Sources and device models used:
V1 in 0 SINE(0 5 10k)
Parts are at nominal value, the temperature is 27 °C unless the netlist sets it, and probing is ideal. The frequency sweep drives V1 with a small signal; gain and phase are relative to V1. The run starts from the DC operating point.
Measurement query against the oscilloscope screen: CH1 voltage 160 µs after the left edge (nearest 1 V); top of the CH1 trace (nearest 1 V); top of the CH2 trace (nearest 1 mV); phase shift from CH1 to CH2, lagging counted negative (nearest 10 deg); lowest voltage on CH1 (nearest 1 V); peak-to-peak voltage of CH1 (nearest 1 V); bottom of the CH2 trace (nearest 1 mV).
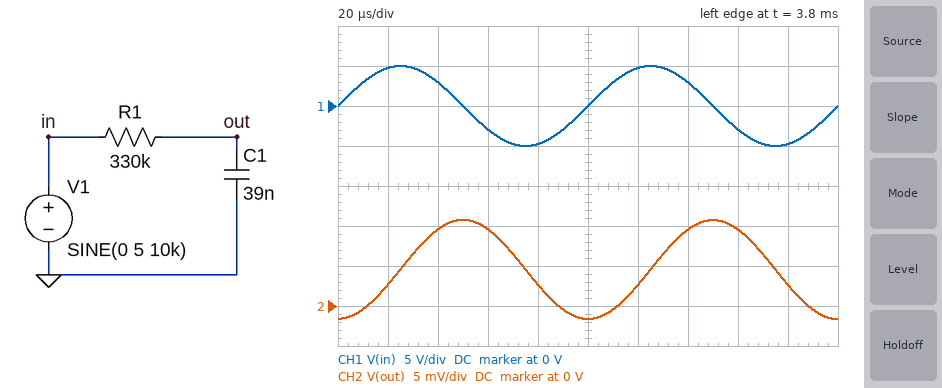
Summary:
-3 V
5 V
11 mV
-90 deg
-5 V
10 V
-2 mV
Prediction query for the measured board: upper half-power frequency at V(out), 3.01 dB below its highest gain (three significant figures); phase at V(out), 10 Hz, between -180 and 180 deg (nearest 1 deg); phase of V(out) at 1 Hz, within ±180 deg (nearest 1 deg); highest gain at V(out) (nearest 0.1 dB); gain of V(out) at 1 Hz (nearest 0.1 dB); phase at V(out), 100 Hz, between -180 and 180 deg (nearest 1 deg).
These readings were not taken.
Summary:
12.4 Hz
-39 deg
-5 deg
0 dB
0 dB
-83 deg
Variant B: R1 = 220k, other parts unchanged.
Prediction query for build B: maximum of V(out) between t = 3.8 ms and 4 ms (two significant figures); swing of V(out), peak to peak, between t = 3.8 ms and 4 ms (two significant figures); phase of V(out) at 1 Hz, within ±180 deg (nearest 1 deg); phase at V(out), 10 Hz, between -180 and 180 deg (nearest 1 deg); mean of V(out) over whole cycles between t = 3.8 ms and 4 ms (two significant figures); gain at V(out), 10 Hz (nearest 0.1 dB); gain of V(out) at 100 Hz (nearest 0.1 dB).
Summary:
15 mV
19 mV
-3 deg
-28 deg
5.9 mV
-1.1 dB
-14.8 dB
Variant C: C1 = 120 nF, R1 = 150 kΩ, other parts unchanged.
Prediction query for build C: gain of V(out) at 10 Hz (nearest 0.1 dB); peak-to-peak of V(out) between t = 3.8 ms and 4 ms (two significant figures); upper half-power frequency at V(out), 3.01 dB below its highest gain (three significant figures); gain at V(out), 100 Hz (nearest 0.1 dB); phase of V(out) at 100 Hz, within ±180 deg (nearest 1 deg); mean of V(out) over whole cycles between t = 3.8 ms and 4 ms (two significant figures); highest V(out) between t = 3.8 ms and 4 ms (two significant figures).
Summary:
-3.6 dB
8.9 mV
8.84 Hz
-21.1 dB
-85 deg
3.6 mV
8.0 mV
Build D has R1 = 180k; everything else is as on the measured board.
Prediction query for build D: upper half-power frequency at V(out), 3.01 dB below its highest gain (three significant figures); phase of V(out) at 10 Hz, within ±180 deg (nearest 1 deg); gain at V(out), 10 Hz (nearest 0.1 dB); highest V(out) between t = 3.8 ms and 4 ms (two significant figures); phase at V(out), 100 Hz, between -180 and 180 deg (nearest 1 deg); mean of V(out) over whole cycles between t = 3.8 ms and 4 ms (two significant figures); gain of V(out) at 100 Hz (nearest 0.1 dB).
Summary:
22.7 Hz
-24 deg
-0.8 dB
18 mV
-77 deg
6.5 mV
-13.1 dB
